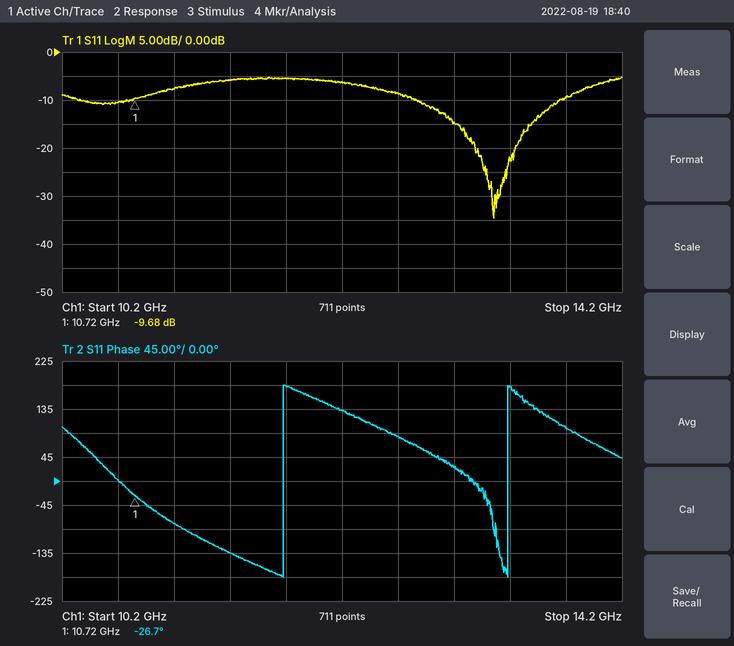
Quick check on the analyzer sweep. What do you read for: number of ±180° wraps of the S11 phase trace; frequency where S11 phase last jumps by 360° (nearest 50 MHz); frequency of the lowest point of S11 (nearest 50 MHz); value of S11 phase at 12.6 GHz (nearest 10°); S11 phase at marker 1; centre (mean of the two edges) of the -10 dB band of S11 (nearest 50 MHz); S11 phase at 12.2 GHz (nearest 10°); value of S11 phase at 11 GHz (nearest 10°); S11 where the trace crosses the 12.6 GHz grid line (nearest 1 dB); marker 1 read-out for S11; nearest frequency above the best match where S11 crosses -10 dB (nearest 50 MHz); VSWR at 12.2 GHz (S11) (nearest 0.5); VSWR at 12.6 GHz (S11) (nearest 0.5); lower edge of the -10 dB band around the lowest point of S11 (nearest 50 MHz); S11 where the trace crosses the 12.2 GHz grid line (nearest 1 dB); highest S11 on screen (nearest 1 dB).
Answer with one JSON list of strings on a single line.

["2", "13.40 GHz", "13.30 GHz", "80°", "-26.7°", "13.25 GHz", "130°", "-80°", "-9 dB", "-9.68 dB", "13.75 GHz", "3.0", "2.0", "12.75 GHz", "-6 dB", "-5 dB"]
